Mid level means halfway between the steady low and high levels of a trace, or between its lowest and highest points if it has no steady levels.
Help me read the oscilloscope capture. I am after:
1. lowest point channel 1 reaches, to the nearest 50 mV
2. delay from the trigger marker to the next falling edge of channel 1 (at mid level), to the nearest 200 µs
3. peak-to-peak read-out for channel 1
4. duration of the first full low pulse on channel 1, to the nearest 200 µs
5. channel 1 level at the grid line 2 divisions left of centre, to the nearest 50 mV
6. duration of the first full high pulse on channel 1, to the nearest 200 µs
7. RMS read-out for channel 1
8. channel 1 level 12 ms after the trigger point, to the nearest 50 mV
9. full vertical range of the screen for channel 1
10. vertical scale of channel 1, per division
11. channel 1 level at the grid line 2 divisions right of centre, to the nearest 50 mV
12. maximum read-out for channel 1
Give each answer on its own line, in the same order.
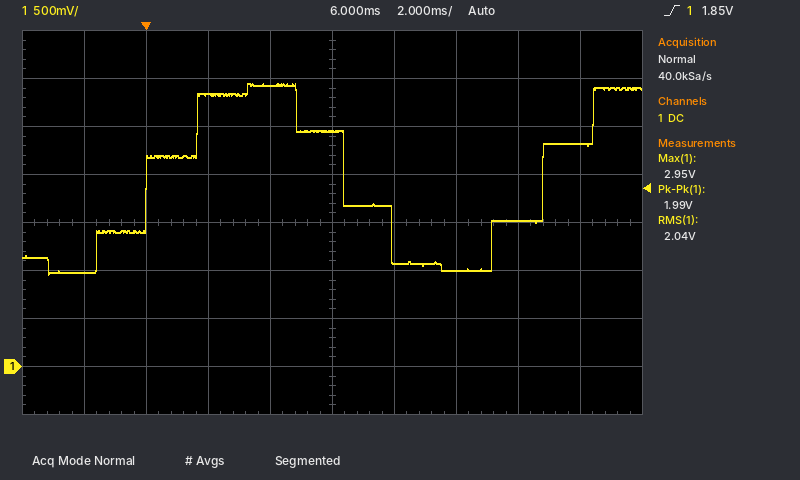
950 mV
6.4 ms
1.99 V
6.4 ms
2.85 V
6.4 ms
2.04 V
1.50 V
4 V
500 mV
1.00 V
2.95 V
